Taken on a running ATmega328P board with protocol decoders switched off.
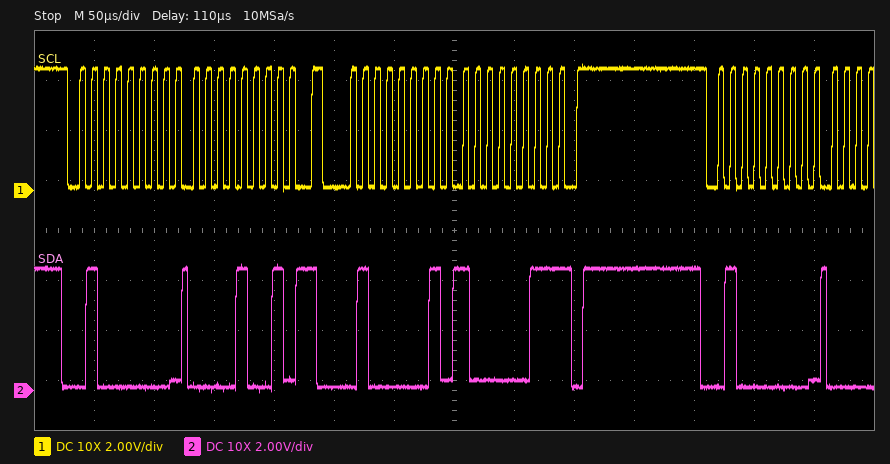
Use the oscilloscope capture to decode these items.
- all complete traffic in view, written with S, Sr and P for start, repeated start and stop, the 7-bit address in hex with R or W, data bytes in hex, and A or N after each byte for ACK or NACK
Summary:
S 20W A 09 A Sr 20R A 83 N P S 20W A
